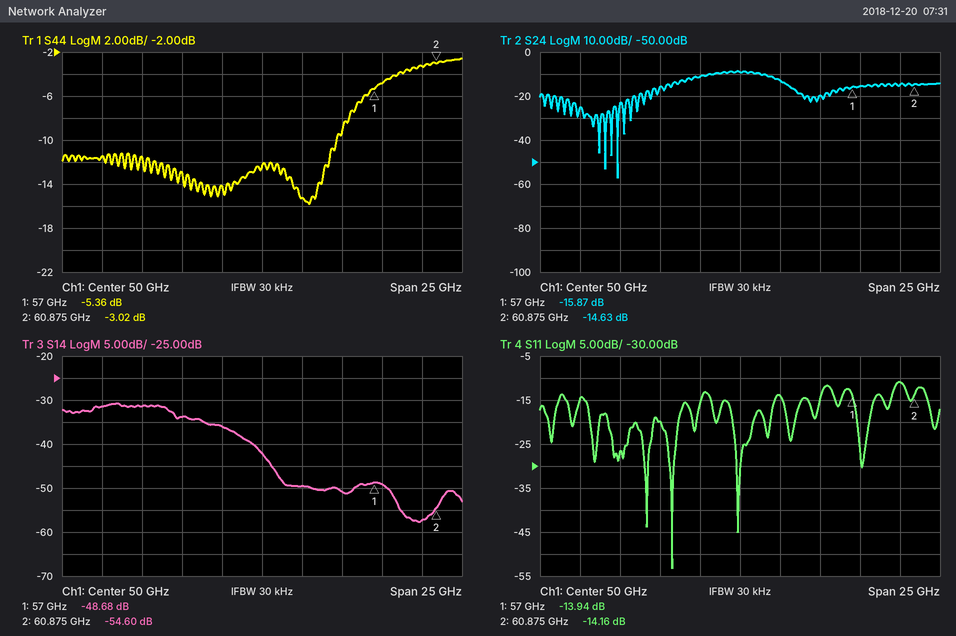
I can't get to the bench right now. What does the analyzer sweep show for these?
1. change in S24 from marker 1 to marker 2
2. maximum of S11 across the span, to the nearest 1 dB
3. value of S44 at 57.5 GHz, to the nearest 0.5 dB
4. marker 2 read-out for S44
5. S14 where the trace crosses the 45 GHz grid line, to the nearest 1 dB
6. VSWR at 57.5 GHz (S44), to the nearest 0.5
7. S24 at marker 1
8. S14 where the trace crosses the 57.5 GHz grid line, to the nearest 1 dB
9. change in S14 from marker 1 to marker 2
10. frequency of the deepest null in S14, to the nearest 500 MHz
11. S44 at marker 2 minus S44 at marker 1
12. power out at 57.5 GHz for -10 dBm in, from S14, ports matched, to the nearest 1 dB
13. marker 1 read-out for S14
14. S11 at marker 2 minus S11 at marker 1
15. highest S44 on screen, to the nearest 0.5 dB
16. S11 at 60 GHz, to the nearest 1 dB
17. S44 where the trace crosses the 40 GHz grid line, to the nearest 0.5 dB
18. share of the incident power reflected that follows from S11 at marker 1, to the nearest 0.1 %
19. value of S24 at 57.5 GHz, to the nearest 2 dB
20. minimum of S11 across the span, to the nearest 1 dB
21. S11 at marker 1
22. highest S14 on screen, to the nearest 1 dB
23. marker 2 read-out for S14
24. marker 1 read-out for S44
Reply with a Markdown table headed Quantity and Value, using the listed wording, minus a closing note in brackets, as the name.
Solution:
| Quantity | Value |
|---|---|
| change in S24 from marker 1 to marker 2 | 1.24 dB |
| maximum of S11 across the span, to the nearest 1 dB | -11 dB |
| value of S44 at 57.5 GHz, to the nearest 0.5 dB | -5.0 dB |
| marker 2 read-out for S44 | -3.02 dB |
| S14 where the trace crosses the 45 GHz grid line, to the nearest 1 dB | -34 dB |
| VSWR at 57.5 GHz (S44), to the nearest 0.5 | 3.5 |
| S24 at marker 1 | -15.87 dB |
| S14 where the trace crosses the 57.5 GHz grid line, to the nearest 1 dB | -49 dB |
| change in S14 from marker 1 to marker 2 | -5.92 dB |
| frequency of the deepest null in S14, to the nearest 500 MHz | 60.0 GHz |
| S44 at marker 2 minus S44 at marker 1 | 2.34 dB |
| power out at 57.5 GHz for -10 dBm in, from S14, ports matched, to the nearest 1 dB | -59 dBm |
| marker 1 read-out for S14 | -48.68 dB |
| S11 at marker 2 minus S11 at marker 1 | -0.22 dB |
| highest S44 on screen, to the nearest 0.5 dB | -2.5 dB |
| S11 at 60 GHz, to the nearest 1 dB | -11 dB |
| S44 where the trace crosses the 40 GHz grid line, to the nearest 0.5 dB | -11.5 dB |
| share of the incident power reflected that follows from S11 at marker 1, to the nearest 0.1 % | 4.0 % |
| value of S24 at 57.5 GHz, to the nearest 2 dB | -16 dB |
| minimum of S11 across the span, to the nearest 1 dB | -53 dB |
| S11 at marker 1 | -13.94 dB |
| highest S14 on screen, to the nearest 1 dB | -31 dB |
| marker 2 read-out for S14 | -54.60 dB |
| marker 1 read-out for S44 | -5.36 dB |
